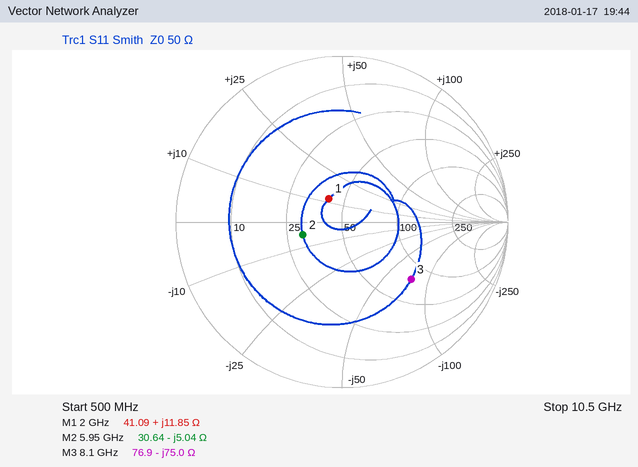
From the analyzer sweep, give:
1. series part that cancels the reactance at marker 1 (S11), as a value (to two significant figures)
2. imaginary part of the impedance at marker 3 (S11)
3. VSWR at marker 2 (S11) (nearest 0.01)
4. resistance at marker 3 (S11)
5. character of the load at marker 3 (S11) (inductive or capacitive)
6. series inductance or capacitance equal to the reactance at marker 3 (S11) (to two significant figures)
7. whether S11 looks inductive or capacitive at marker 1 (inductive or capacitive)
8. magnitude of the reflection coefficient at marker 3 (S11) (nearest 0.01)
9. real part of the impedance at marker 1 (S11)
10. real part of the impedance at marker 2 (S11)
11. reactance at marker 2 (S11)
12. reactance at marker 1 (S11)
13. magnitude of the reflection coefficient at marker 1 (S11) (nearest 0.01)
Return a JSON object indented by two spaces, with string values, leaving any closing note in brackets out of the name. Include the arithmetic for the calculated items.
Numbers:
{
  "series part that cancels the reactance at marker 1 (S11), as a value": "C = 1/(2π × 2 GHz × 11.85 Ω) ≈ 6.7 pF",
  "imaginary part of the impedance at marker 3": "-75.0 Ω",
  "VSWR at marker 2 (S11)": "1.66",
  "resistance at marker 3": "76.9 Ω",
  "character of the load at marker 3 (S11)": "capacitive",
  "series inductance or capacitance equal to the reactance at marker 3 (S11)": "C = 1/(2π × 8.1 GHz × 75 Ω) ≈ 262 fF, so 260 fF to two significant figures",
  "whether S11 looks inductive or capacitive at marker 1": "inductive",
  "magnitude of the reflection coefficient at marker 3 (S11)": "0.54",
  "real part of the impedance at marker 1": "41.09 Ω",
  "real part of the impedance at marker 2": "30.64 Ω",
  "reactance at marker 2": "-5.04 Ω",
  "reactance at marker 1": "+11.85 Ω",
  "magnitude of the reflection coefficient at marker 1 (S11)": "0.16"
}
